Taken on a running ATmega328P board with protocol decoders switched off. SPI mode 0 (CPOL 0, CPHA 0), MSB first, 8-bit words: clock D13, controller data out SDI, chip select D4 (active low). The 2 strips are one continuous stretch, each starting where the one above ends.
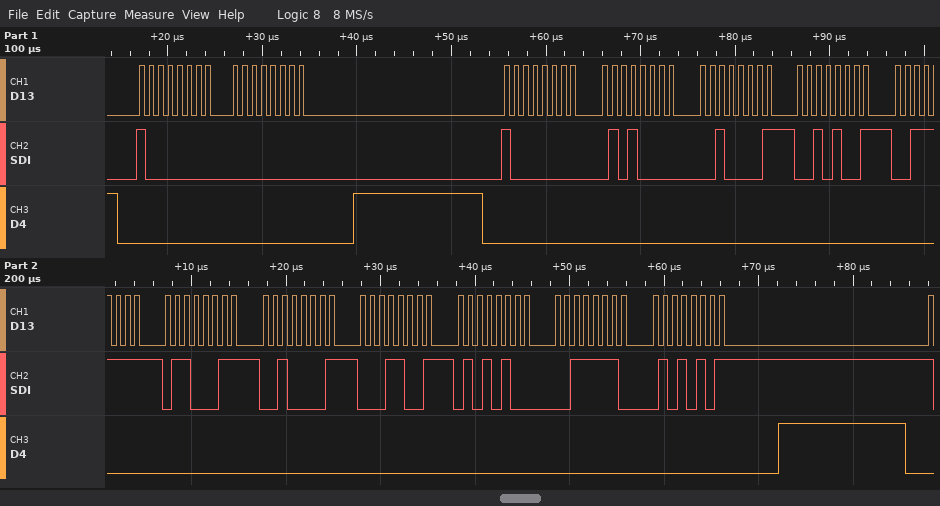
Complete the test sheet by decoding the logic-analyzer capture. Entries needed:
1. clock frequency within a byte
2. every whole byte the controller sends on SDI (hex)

1 MHz
80 00 80 50 21 29 3F 63 21 19 54 3E 55
